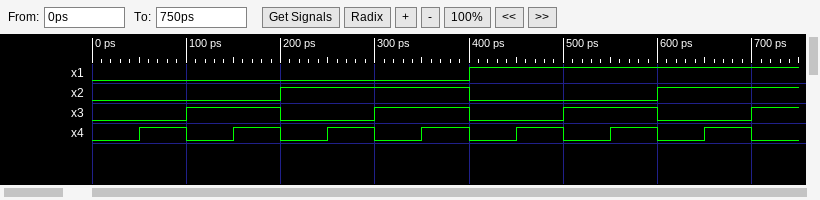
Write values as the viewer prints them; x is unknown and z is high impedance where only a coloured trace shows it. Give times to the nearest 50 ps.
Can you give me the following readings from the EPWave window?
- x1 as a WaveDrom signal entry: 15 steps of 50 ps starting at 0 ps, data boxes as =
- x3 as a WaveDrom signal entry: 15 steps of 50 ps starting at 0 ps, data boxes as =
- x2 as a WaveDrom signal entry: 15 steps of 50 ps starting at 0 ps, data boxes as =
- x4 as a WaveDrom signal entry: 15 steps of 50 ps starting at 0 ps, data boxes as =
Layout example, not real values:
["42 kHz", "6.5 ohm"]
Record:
["{name: 'x1', wave: '0.......1......'}", "{name: 'x3', wave: '0.1.0.1.0.1.0.1'}", "{name: 'x2', wave: '0...1...0...1..'}", "{name: 'x4', wave: '010101010101010'}"]
